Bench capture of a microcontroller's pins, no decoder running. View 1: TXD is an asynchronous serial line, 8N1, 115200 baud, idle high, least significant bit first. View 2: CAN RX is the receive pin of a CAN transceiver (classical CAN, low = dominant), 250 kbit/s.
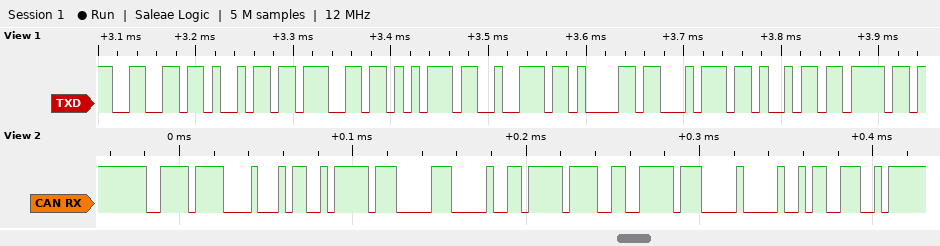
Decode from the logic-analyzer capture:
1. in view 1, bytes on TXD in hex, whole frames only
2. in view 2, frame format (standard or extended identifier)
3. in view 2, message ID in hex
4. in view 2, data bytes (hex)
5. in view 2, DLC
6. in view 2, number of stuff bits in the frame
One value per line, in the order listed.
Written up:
66 69 67 75 72 61 74 69 6F
standard
0x3DE
B2 FF 06 03 7F CC FF 00
8
7
